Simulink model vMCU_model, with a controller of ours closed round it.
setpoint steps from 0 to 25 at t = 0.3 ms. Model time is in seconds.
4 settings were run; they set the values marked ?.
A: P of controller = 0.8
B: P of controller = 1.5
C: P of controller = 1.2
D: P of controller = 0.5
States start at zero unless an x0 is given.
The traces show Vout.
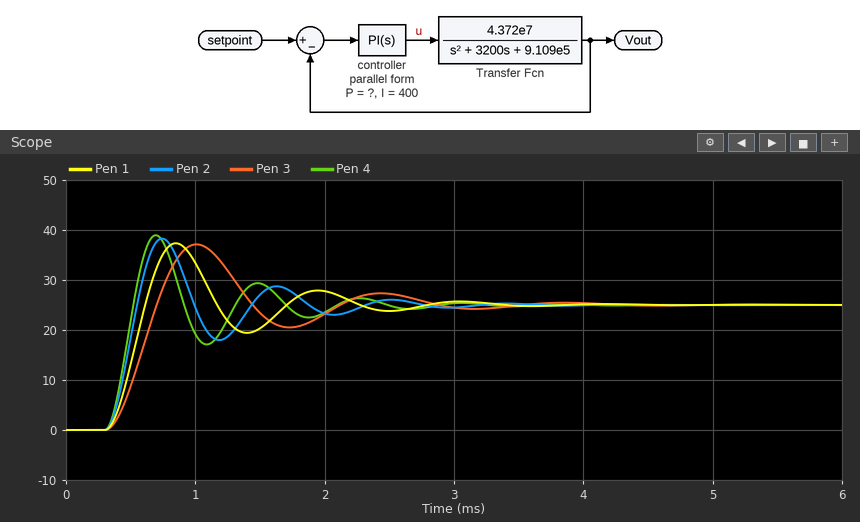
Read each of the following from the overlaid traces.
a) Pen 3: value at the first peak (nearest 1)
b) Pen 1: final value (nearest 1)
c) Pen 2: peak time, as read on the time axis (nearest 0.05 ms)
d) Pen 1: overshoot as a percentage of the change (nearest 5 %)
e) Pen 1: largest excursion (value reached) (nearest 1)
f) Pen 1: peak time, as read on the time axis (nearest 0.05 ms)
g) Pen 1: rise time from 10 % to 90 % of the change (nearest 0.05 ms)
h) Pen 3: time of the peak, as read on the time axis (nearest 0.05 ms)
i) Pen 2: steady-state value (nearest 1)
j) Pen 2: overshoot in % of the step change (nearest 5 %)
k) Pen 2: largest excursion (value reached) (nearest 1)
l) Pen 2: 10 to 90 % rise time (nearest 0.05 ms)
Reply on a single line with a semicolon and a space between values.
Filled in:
37; 25; 0.75 ms; 50 %; 37; 0.85 ms; 0.20 ms; 1.00 ms; 25; 55 %; 38; 0.15 ms
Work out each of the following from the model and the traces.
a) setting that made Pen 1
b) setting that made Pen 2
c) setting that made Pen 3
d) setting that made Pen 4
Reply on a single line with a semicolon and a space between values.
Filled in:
A; C; D; B
